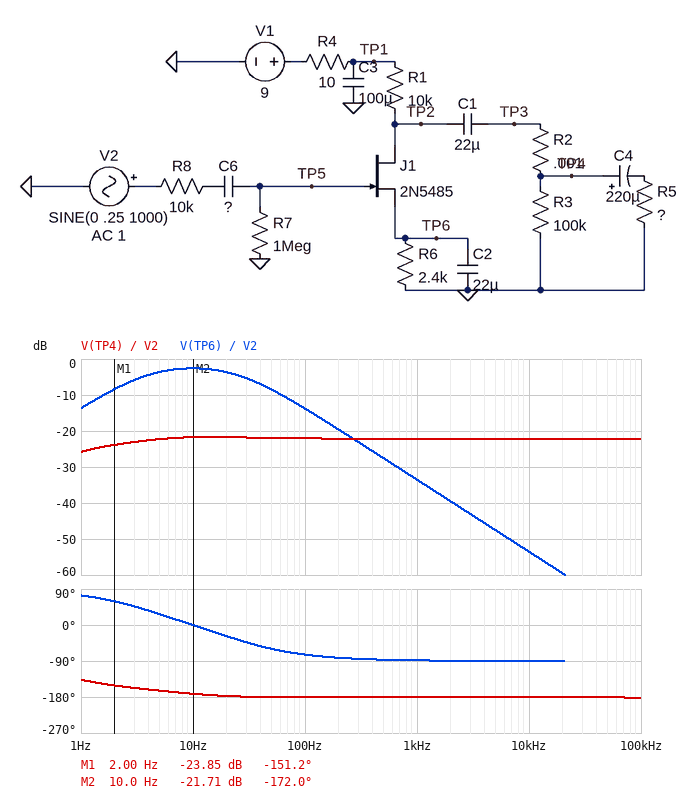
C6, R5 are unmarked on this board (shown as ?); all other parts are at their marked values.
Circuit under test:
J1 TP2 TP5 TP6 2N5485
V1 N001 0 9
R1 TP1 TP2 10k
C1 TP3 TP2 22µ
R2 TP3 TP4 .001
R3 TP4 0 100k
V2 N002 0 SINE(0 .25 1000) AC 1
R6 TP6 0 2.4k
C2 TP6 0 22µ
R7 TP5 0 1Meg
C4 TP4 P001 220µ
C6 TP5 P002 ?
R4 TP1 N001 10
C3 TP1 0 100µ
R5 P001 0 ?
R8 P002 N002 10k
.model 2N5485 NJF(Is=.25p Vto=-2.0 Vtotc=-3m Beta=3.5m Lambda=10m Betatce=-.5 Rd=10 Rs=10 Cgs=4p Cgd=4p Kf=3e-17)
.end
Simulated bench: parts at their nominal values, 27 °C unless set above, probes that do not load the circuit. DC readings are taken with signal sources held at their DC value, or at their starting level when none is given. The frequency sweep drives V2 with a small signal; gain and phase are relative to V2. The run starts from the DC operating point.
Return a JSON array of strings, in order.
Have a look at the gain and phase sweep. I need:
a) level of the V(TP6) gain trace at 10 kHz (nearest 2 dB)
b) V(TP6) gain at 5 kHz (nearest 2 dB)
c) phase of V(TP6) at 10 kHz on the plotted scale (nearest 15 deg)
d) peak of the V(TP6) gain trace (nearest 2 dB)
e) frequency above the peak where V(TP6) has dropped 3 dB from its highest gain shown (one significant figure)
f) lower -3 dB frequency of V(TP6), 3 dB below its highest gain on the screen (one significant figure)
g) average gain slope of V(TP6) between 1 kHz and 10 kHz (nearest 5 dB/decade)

["-54 dB", "-48 dB", "-90 deg", "-2 dB", "30 Hz", "3 Hz", "-20 dB/decade"]
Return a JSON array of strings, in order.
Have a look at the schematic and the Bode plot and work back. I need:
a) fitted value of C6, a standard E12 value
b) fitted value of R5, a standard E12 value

["39 nF", "27 Ω"]
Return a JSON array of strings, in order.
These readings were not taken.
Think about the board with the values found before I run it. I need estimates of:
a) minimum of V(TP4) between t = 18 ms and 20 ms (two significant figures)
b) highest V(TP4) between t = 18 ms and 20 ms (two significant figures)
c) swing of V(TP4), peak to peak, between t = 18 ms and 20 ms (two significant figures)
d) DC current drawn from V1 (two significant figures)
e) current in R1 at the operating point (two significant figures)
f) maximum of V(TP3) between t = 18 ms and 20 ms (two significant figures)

["-25 mV", "12 mV", "37 mV", "650 µA", "650 µA", "12 mV"]
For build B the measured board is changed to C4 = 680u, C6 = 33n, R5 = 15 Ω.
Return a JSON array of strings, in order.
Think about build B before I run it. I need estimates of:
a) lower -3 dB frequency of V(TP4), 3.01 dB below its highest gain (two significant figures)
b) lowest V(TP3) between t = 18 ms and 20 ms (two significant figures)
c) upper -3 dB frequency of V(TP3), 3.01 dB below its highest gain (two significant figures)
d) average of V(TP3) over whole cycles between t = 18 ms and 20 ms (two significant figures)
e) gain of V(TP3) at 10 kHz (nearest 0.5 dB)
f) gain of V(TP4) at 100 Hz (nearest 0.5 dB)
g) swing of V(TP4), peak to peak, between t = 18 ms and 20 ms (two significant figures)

["13 Hz", "-13 mV", "3.4 MHz", "-1.3 mV", "-27.0 dB", "-27.5 dB", "20 mV"]
